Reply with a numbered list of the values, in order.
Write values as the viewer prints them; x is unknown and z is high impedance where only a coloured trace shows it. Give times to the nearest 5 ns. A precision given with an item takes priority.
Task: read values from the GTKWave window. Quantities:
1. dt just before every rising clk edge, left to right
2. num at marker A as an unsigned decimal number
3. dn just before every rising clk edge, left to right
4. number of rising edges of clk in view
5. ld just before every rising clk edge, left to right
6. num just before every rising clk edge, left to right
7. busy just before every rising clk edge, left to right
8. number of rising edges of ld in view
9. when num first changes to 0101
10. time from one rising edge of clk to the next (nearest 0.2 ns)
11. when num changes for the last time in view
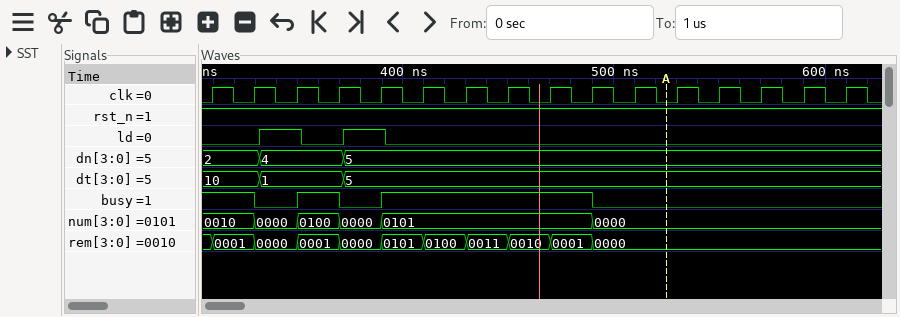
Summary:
1. 10, 10, 1, 1, 5, 5, 5, 5, 5, 5, 5, 5, 5, 5, 5, 5
2. 0
3. 2, 2, 4, 4, 5, 5, 5, 5, 5, 5, 5, 5, 5, 5, 5, 5
4. 16
5. 0 0 1 0 1 0 0 0 0 0 0 0 0 0 0 0
6. 0010, 0010, 0000, 0100, 0000, 0101, 0101, 0101, 0101, 0101, 0000, 0000, 0000, 0000, 0000, 0000
7. 1 1 0 1 0 1 1 1 1 1 0 0 0 0 0 0
8. 2
9. 390 ns
10. 20 ns
11. 490 ns
